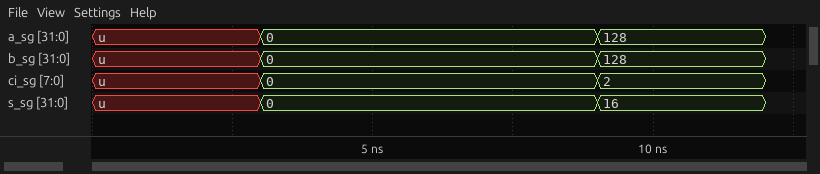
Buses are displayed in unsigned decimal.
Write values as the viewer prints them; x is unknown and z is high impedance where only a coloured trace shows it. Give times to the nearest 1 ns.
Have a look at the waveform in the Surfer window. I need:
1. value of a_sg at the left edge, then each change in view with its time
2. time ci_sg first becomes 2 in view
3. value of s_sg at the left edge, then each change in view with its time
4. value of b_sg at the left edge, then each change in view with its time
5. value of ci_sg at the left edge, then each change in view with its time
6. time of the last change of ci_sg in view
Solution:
u, 0 at 3 ns, 128 at 9 ns
9 ns
u, 0 at 3 ns, 16 at 9 ns
u, 0 at 3 ns, 128 at 9 ns
u, 0 at 3 ns, 2 at 9 ns
9 ns
